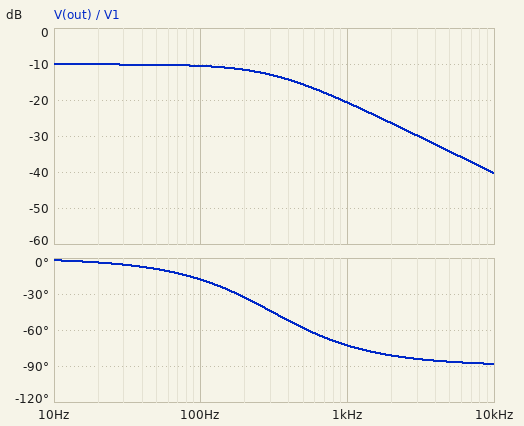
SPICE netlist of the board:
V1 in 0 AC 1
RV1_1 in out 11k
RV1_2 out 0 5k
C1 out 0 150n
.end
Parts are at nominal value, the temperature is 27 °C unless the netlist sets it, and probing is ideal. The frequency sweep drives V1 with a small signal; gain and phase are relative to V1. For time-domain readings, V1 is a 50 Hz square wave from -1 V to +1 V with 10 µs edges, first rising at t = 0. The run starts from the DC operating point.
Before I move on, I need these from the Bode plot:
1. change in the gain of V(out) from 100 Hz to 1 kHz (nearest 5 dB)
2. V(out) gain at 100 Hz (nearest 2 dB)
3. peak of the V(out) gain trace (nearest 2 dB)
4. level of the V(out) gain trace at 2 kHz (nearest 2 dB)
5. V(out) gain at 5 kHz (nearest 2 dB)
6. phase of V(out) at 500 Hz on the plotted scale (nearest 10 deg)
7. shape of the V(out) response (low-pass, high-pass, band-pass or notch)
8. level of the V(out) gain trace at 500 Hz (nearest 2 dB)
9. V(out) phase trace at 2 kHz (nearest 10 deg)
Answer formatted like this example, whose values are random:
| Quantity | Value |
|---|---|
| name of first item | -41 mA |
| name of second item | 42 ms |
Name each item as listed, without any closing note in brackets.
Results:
| Quantity | Value |
|---|---|
| change in the gain of V(out) from 100 Hz to 1 kHz | -10 dB |
| V(out) gain at 100 Hz | -10 dB |
| peak of the V(out) gain trace | -10 dB |
| level of the V(out) gain trace at 2 kHz | -26 dB |
| V(out) gain at 5 kHz | -34 dB |
| phase of V(out) at 500 Hz on the plotted scale | -60 deg |
| shape of the V(out) response | low-pass |
| level of the V(out) gain trace at 500 Hz | -16 dB |
| V(out) phase trace at 2 kHz | -80 deg |
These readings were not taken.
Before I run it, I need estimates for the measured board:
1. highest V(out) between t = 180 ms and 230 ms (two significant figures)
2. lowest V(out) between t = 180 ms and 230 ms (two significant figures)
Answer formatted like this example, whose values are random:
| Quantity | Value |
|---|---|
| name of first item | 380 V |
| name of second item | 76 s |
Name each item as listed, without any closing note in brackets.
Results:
| Quantity | Value |
|---|---|
| highest V(out) between t = 180 ms and 230 ms | 310 mV |
| lowest V(out) between t = 180 ms and 230 ms | -310 mV |
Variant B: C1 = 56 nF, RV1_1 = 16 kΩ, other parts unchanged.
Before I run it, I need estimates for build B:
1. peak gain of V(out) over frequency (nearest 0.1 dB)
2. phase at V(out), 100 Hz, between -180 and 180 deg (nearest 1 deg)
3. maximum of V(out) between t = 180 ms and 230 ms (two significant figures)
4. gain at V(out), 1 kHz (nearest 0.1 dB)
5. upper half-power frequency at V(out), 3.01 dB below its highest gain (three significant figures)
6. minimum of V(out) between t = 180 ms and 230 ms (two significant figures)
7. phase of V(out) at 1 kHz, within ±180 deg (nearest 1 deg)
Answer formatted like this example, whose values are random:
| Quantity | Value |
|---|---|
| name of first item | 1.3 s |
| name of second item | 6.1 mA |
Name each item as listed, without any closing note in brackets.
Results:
| Quantity | Value |
|---|---|
| peak gain of V(out) over frequency | -12.5 dB |
| phase at V(out), 100 Hz, between -180 and 180 deg | -8 deg |
| maximum of V(out) between t = 180 ms and 230 ms | 240 mV |
| gain at V(out), 1 kHz | -16.9 dB |
| upper half-power frequency at V(out), 3.01 dB below its highest gain | 746 Hz |
| minimum of V(out) between t = 180 ms and 230 ms | -240 mV |
| phase of V(out) at 1 kHz, within ±180 deg | -53 deg |
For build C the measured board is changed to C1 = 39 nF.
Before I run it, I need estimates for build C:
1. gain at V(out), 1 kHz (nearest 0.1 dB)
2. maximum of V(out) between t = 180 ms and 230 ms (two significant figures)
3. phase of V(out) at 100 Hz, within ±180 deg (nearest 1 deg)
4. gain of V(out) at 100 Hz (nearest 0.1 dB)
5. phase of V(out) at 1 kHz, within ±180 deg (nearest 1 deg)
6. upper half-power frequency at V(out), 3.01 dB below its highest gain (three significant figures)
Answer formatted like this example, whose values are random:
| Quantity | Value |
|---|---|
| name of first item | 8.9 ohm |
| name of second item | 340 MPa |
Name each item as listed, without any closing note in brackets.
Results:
| Quantity | Value |
|---|---|
| gain at V(out), 1 kHz | -12.4 dB |
| maximum of V(out) between t = 180 ms and 230 ms | 310 mV |
| phase of V(out) at 100 Hz, within ±180 deg | -5 deg |
| gain of V(out) at 100 Hz | -10.1 dB |
| phase of V(out) at 1 kHz, within ±180 deg | -40 deg |
| upper half-power frequency at V(out), 3.01 dB below its highest gain | 1.19 kHz |
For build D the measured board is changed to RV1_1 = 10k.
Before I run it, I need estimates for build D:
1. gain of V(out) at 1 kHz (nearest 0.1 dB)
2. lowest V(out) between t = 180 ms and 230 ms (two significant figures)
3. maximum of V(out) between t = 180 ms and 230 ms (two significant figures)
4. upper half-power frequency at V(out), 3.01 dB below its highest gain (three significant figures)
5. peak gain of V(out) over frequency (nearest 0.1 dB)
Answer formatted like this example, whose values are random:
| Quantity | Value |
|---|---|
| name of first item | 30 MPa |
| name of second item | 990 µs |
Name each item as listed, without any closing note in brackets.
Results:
| Quantity | Value |
|---|---|
| gain of V(out) at 1 kHz | -19.9 dB |
| lowest V(out) between t = 180 ms and 230 ms | -330 mV |
| maximum of V(out) between t = 180 ms and 230 ms | 330 mV |
| upper half-power frequency at V(out), 3.01 dB below its highest gain | 318 Hz |
| peak gain of V(out) over frequency | -9.5 dB |
